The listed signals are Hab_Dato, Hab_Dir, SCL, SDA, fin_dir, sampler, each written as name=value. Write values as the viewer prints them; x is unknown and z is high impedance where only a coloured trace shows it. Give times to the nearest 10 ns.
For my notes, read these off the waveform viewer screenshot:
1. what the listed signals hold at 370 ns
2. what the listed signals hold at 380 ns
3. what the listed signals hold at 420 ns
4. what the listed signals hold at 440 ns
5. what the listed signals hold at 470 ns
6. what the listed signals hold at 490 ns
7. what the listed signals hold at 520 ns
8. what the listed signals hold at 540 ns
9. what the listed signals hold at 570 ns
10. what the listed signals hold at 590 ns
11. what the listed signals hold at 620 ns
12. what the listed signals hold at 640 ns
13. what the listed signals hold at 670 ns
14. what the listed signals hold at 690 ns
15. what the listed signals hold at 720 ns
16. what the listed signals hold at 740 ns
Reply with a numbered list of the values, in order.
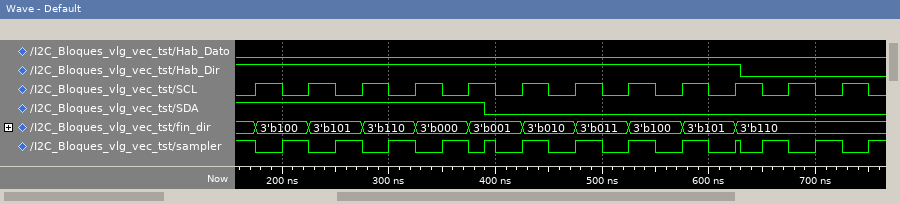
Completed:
1. Hab_Dato=0, Hab_Dir=1, SCL=0, SDA=1, fin_dir=3'b000, sampler=1
2. Hab_Dato=0, Hab_Dir=1, SCL=1, SDA=1, fin_dir=3'b001, sampler=0
3. Hab_Dato=0, Hab_Dir=1, SCL=0, SDA=0, fin_dir=3'b001, sampler=0
4. Hab_Dato=0, Hab_Dir=1, SCL=1, SDA=0, fin_dir=3'b010, sampler=1
5. Hab_Dato=0, Hab_Dir=1, SCL=0, SDA=0, fin_dir=3'b010, sampler=0
6. Hab_Dato=0, Hab_Dir=1, SCL=1, SDA=0, fin_dir=3'b011, sampler=1
7. Hab_Dato=0, Hab_Dir=1, SCL=0, SDA=0, fin_dir=3'b011, sampler=0
8. Hab_Dato=0, Hab_Dir=1, SCL=1, SDA=0, fin_dir=3'b100, sampler=1
9. Hab_Dato=0, Hab_Dir=1, SCL=0, SDA=0, fin_dir=3'b100, sampler=0
10. Hab_Dato=0, Hab_Dir=1, SCL=1, SDA=0, fin_dir=3'b101, sampler=1
11. Hab_Dato=0, Hab_Dir=1, SCL=0, SDA=0, fin_dir=3'b101, sampler=0
12. Hab_Dato=0, Hab_Dir=0, SCL=1, SDA=0, fin_dir=3'b110, sampler=0
13. Hab_Dato=0, Hab_Dir=0, SCL=0, SDA=0, fin_dir=3'b110, sampler=1
14. Hab_Dato=0, Hab_Dir=0, SCL=1, SDA=0, fin_dir=3'b110, sampler=0
15. Hab_Dato=0, Hab_Dir=0, SCL=0, SDA=0, fin_dir=3'b110, sampler=1
16. Hab_Dato=0, Hab_Dir=0, SCL=1, SDA=0, fin_dir=3'b110, sampler=0
